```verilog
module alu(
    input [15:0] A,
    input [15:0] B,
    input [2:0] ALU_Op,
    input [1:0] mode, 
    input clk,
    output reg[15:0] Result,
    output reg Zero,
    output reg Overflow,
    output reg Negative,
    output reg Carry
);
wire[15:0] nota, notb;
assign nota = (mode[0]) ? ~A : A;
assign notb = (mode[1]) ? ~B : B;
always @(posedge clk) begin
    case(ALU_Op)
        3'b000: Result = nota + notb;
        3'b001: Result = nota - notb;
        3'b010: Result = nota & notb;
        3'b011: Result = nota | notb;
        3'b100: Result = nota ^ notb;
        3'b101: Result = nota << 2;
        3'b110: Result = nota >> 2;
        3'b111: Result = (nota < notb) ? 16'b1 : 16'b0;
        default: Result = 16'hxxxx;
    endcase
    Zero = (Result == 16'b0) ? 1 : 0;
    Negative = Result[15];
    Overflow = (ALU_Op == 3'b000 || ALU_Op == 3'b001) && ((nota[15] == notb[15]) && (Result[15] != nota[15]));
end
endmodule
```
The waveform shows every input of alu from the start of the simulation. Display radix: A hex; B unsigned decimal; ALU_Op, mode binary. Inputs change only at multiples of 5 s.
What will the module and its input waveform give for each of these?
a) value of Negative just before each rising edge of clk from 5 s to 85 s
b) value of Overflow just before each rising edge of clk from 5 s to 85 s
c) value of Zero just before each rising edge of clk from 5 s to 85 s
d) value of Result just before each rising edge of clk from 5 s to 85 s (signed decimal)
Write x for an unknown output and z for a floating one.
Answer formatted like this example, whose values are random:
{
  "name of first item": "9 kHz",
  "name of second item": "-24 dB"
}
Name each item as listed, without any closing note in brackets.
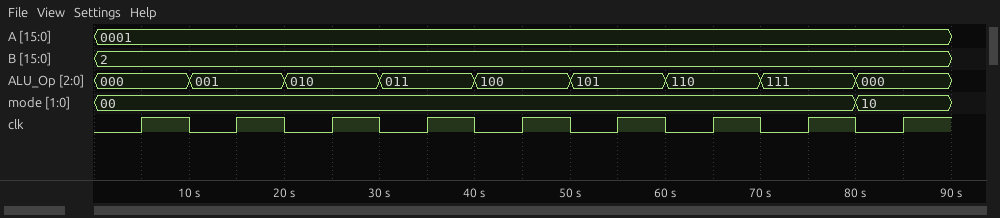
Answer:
{
  "value of Negative just before each rising edge of clk from 5 s to 85 s": "x 0 1 0 0 0 0 0 0",
  "value of Overflow just before each rising edge of clk from 5 s to 85 s": "x 0 1 0 0 0 0 0 0",
  "value of Zero just before each rising edge of clk from 5 s to 85 s": "x 0 0 1 0 0 0 1 0",
  "value of Result just before each rising edge of clk from 5 s to 85 s": "x, 3, -1, 0, 3, 3, 4, 0, 1"
}
